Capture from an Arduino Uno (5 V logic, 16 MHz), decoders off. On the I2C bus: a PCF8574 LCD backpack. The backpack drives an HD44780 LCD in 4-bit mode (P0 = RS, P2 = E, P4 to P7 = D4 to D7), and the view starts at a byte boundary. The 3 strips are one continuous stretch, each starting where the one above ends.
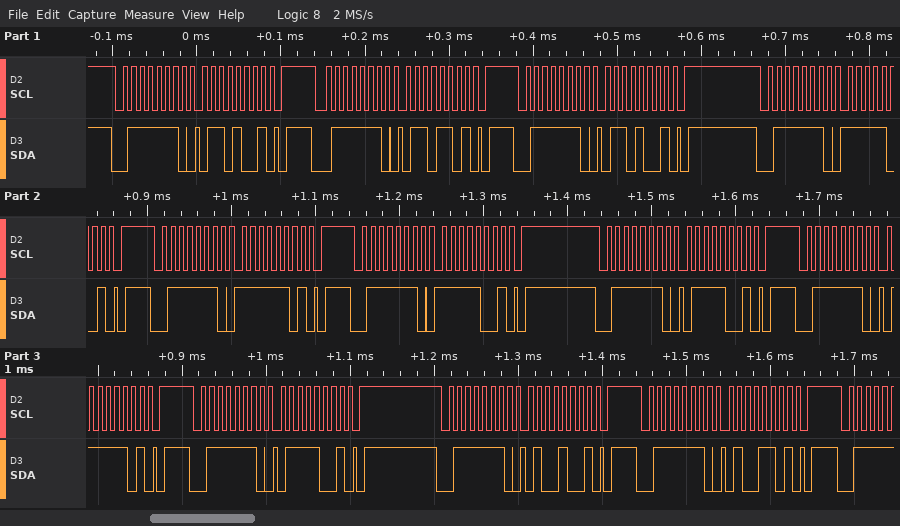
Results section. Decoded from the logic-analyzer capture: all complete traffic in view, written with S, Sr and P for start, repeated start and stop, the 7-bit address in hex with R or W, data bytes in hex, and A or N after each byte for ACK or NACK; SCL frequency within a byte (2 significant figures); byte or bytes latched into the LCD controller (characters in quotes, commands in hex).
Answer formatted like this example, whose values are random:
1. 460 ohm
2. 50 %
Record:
1. S 3FW A 69 A P S 3FW A 6D A P S 3FW A 69 A P S 3FW A F9 A P S 3FW A FD A P S 3FW A F9 A P S 3FW A 79 A P S 3FW A 7D A P S 3FW A 79 A P S 3FW A 49 A P S 3FW A 4D A P
2. 100 kHz
3. 'o'
